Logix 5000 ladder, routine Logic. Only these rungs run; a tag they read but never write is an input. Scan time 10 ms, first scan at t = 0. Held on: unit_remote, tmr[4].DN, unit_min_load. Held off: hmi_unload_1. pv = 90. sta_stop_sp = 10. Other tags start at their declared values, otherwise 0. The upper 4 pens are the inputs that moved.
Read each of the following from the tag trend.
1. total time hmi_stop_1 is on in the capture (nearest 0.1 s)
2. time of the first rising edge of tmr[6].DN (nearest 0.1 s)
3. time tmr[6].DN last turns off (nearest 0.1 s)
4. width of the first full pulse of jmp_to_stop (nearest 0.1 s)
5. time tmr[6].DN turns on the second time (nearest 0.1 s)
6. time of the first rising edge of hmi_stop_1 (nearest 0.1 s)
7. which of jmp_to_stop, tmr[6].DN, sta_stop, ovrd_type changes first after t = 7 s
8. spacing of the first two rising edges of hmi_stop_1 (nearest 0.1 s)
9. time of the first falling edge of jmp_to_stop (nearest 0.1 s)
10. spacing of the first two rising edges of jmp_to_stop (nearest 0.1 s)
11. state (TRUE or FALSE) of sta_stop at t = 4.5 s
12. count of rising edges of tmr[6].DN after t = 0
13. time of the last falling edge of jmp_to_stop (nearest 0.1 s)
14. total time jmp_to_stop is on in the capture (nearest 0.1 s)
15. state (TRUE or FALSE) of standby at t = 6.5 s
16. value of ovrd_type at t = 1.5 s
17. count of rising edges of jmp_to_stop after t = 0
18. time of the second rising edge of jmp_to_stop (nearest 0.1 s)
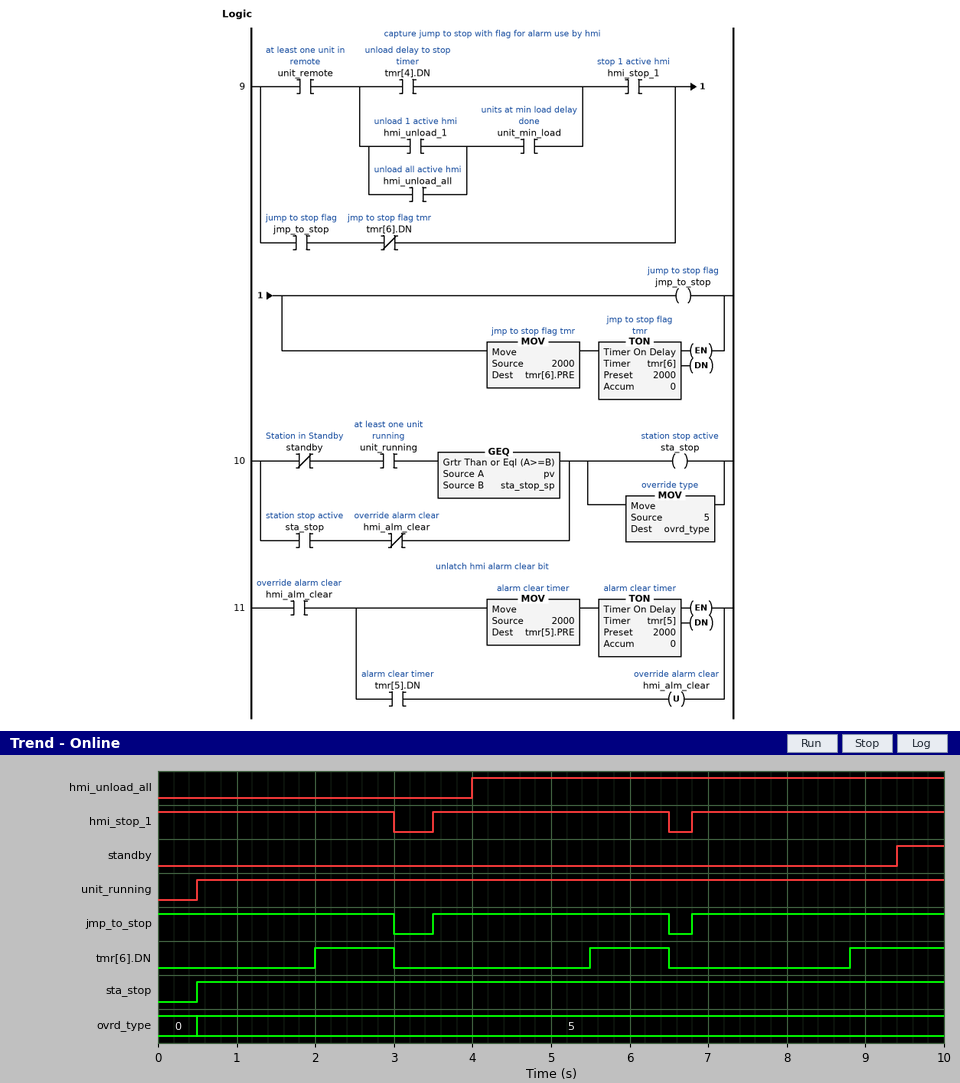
9.2 s
2.0 s
6.5 s
3.0 s
5.5 s
3.5 s
tmr[6].DN
3.3 s
3.0 s
3.3 s
TRUE
3
6.5 s
9.2 s
FALSE
5
2
6.8 s
